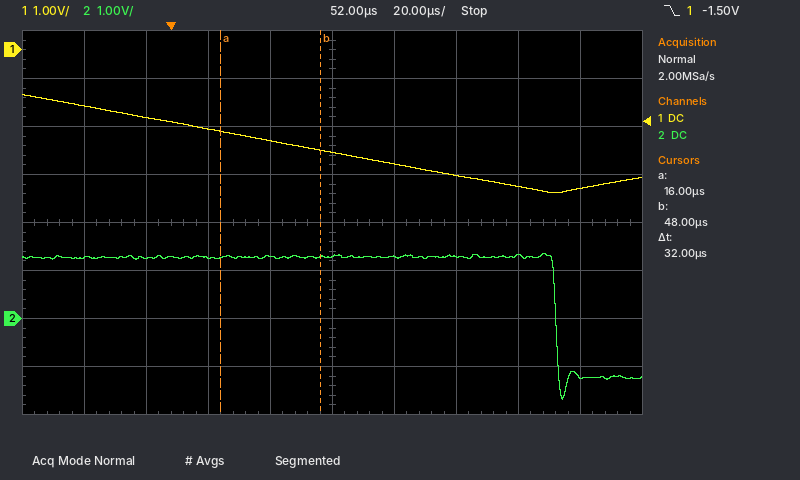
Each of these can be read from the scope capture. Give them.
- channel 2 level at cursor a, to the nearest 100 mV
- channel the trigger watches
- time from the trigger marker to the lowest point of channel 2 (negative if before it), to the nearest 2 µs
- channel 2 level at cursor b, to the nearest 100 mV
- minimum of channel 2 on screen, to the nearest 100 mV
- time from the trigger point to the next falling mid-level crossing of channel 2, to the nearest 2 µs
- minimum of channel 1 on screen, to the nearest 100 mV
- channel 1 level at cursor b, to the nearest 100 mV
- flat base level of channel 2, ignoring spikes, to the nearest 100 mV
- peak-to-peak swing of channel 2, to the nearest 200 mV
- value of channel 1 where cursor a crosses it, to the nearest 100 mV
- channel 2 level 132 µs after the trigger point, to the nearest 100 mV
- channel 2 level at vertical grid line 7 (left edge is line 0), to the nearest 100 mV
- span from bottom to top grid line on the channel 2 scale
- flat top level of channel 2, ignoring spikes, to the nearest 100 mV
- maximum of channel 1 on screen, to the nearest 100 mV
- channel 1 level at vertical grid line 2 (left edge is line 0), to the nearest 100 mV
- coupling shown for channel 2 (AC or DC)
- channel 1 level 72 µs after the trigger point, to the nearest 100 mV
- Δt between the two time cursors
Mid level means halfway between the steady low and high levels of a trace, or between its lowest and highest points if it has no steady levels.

1.3 V
channel 1
+126 µs
1.3 V
-1.7 V
124 µs
-3.0 V
-2.1 V
-1.2 V
3.0 V
-1.7 V
-1.2 V
1.3 V
8 V
1.3 V
-900 mV
-1.4 V
DC
-2.4 V
32 µs
